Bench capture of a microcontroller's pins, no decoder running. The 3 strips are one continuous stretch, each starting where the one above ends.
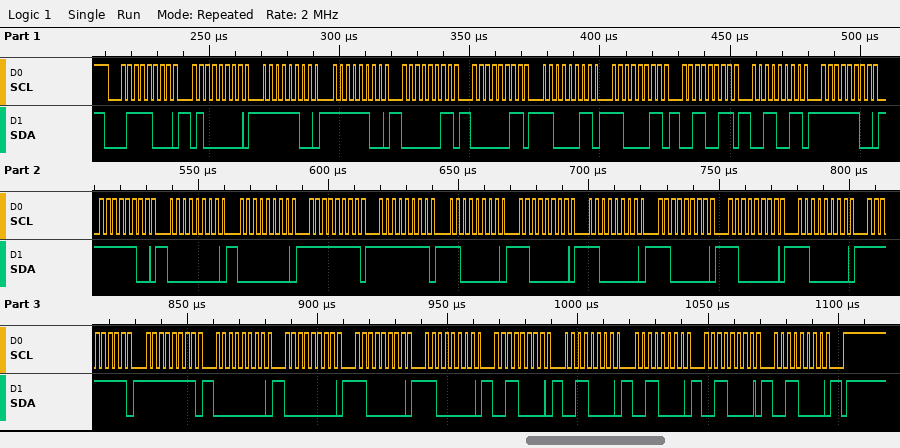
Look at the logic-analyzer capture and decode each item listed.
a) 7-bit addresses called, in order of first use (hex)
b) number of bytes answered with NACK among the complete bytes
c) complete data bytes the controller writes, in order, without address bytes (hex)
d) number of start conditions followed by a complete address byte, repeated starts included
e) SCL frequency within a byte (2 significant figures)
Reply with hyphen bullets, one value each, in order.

- 0x3C
- 0
- 40 FC FC 03 03 C3 C3 33 33 FC FC 00 00 FF FF C0 C0 C0 C0 C0 C0 FF FF 00 00 C0 C0 30 30 30 30 30
- 1
- 400 kHz
